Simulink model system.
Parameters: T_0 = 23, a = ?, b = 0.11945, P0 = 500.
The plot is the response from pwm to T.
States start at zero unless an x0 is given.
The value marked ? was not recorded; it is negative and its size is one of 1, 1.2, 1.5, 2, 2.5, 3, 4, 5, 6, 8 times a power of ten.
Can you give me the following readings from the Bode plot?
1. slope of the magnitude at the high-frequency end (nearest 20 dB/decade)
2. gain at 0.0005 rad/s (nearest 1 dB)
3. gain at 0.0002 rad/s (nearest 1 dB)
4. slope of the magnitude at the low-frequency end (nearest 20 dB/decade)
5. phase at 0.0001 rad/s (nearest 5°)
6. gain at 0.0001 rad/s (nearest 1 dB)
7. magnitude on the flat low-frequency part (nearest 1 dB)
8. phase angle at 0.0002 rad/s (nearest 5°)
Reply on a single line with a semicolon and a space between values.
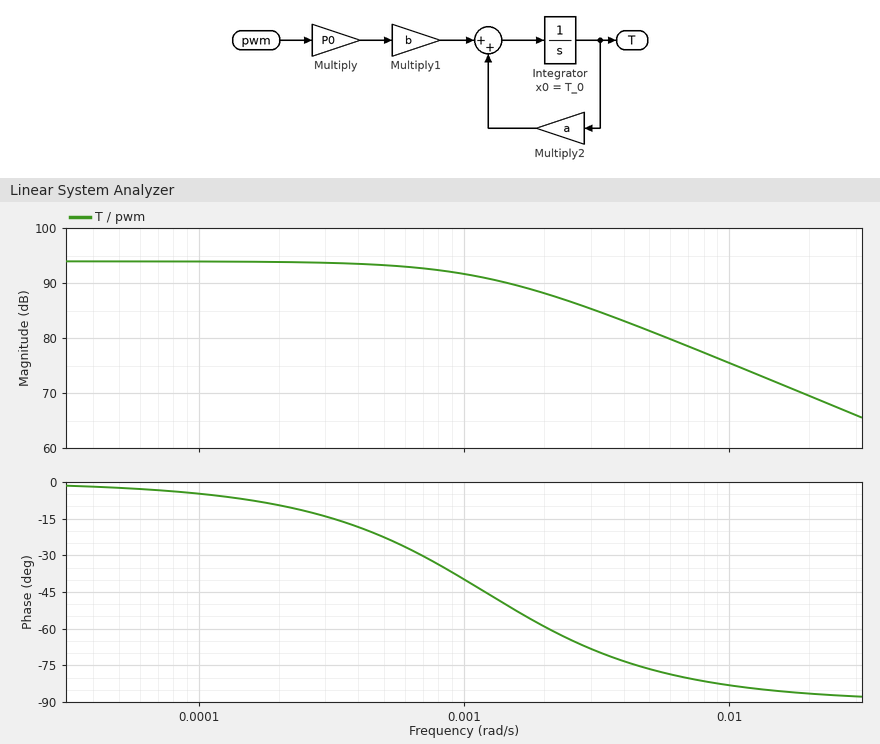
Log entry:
-20 dB/decade; 93 dB; 94 dB; 0 dB/decade; -5°; 94 dB; 94 dB; -10°
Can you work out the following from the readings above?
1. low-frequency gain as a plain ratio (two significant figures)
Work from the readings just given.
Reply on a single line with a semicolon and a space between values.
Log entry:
50000
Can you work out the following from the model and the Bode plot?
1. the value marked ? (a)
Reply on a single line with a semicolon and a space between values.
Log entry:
-0.0012
